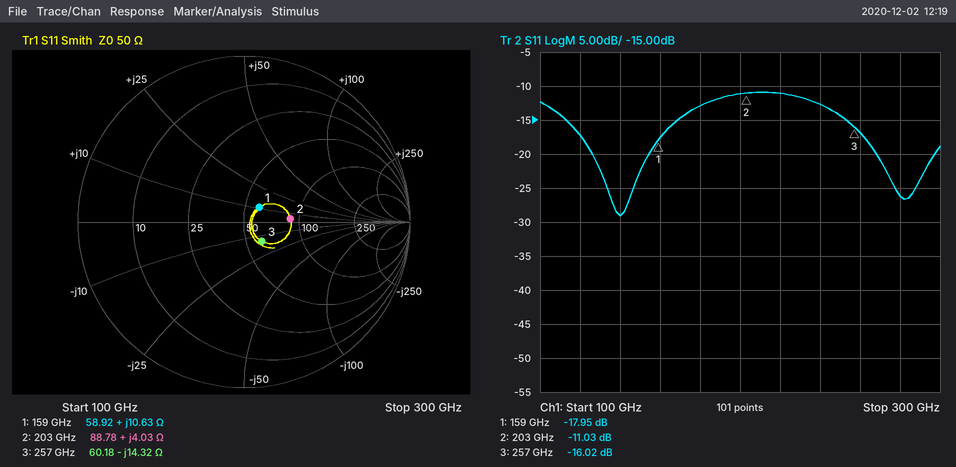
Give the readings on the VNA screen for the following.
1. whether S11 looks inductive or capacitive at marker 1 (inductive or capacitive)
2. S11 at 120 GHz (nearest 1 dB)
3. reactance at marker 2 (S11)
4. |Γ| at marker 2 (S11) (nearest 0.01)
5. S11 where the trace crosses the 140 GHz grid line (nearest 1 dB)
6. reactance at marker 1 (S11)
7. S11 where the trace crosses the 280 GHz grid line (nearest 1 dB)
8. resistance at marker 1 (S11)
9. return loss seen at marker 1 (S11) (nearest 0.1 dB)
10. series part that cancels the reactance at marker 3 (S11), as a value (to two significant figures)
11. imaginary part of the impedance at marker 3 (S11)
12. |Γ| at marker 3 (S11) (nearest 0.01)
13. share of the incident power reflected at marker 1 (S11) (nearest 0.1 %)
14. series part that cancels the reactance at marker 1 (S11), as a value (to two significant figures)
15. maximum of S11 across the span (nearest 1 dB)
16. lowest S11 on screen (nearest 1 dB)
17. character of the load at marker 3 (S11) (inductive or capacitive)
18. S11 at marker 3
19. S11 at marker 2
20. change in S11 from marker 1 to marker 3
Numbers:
inductive
-17 dB
+4.03 Ω
0.28
-29 dB
+10.63 Ω
-26 dB
58.92 Ω
17.9 dB
8.9 pH
-14.32 Ω
0.16
1.6 %
94 fF
-11 dB
-29 dB
capacitive
-16.02 dB
-11.03 dB
1.93 dB
